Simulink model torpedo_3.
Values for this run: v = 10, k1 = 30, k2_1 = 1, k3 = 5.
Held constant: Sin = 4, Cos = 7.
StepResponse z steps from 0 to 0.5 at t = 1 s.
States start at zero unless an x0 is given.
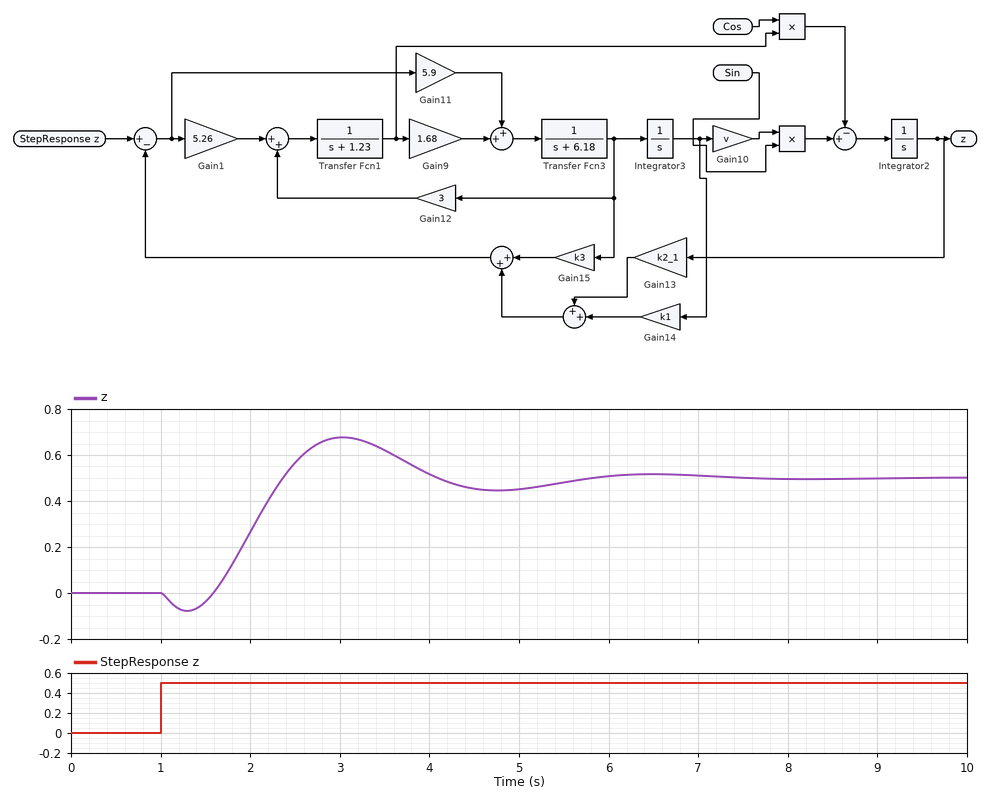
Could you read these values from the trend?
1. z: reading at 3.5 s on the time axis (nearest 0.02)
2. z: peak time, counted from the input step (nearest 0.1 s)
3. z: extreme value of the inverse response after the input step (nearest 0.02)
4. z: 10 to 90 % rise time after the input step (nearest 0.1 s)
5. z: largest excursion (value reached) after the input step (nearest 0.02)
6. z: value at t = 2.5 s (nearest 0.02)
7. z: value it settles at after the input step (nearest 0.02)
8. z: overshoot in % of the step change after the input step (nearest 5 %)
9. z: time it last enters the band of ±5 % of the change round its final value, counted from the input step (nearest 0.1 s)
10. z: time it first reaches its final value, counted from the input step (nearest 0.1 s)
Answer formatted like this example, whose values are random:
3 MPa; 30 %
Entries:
0.62; 2.0 s; -0.08; 0.6 s; 0.68; 0.56; 0.50; 35 %; 4.4 s; 1.4 s
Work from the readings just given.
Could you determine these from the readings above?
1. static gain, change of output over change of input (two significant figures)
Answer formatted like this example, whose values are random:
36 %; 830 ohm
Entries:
1.0
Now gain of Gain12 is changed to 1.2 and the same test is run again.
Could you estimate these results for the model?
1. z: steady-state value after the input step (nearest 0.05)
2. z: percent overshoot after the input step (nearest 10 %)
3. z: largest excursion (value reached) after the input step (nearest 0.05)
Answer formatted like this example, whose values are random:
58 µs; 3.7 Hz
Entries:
0.50; 20 %; 0.60
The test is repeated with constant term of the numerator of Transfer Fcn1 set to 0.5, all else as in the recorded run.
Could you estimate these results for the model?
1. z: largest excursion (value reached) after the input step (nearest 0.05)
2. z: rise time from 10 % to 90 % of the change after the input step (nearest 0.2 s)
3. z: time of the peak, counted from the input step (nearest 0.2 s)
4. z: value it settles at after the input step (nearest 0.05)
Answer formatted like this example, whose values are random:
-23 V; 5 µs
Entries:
0.55; 1.0 s; 2.2 s; 0.50
